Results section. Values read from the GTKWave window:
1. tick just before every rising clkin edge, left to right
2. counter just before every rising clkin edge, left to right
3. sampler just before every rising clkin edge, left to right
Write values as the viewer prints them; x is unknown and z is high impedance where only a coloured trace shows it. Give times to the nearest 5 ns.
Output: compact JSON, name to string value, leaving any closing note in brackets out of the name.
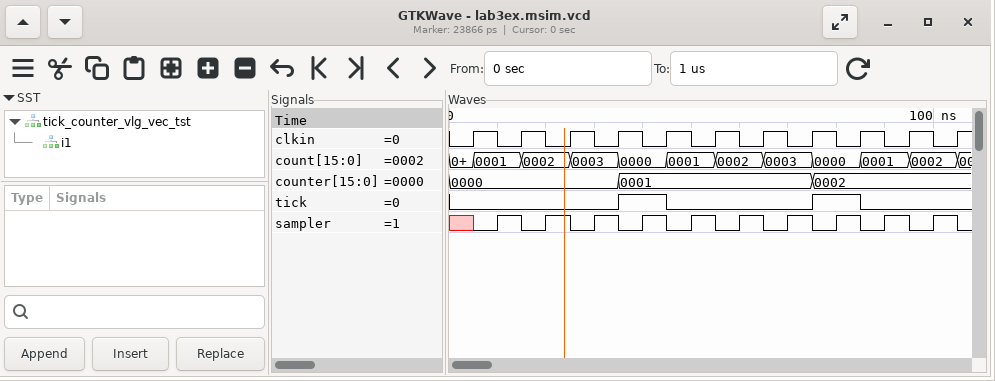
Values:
{"tick just before every rising clkin edge, left to right": "0 0 0 0 1 0 0 0 1 0 0", "counter just before every rising clkin edge, left to right": "0000, 0000, 0000, 0000, 0001, 0001, 0001, 0001, 0002, 0002, 0002", "sampler just before every rising clkin edge, left to right": "x 1 1 1 1 1 1 1 1 1 1"}
